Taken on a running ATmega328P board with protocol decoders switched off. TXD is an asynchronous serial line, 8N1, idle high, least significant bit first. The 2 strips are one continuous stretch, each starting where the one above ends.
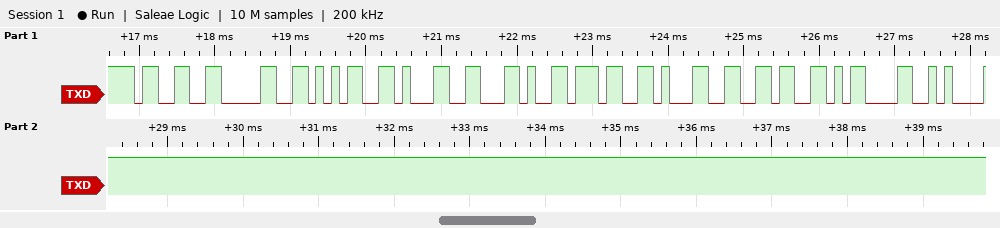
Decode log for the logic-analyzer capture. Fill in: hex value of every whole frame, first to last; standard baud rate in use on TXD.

0x33 0x30 0x35 0x31 0x2C 0x37 0x31 0x36 0x0D 0x0A
9600 baud
